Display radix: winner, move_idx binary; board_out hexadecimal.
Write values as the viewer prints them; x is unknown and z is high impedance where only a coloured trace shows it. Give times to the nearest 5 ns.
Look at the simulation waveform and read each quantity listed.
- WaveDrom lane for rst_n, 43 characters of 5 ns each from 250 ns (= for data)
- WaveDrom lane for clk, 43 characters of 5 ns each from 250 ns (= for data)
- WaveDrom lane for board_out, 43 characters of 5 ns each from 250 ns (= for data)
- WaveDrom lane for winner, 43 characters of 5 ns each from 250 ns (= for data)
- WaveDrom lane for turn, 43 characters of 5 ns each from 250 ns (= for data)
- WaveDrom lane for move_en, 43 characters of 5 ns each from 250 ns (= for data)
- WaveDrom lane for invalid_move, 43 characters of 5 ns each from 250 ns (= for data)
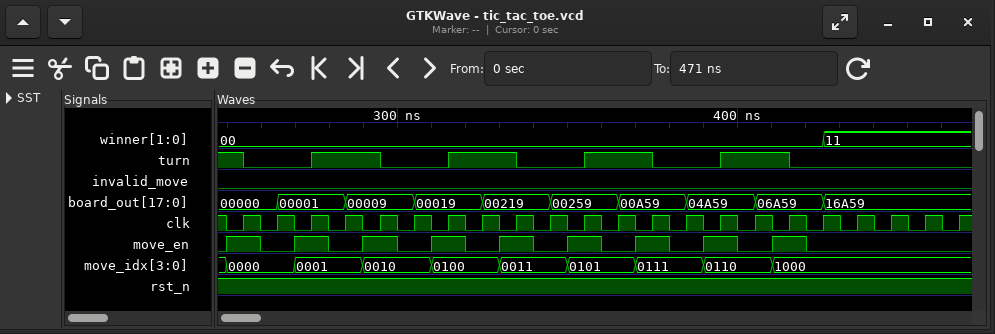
{name: 'rst_n', wave: '1..........................................'}
{name: 'clk', wave: '0101010101010101010101010101010101010101010'}
{name: 'board_out', wave: '=..=...=...=...=...=...=...=...=...=.......', data: '00000 00001 00009 00019 00219 00259 00A59 04A59 06A59 16A59'}
{name: 'winner', wave: '=..................................=.......', data: '00 11'}
{name: 'turn', wave: '10...1...0...1...0...1...0...1...0.........'}
{name: 'move_en', wave: '1.0.1.0.1.0.1.0.1.0.1.0.1.0.1.0.1.0........'}
{name: 'invalid_move', wave: '0..........................................'}
